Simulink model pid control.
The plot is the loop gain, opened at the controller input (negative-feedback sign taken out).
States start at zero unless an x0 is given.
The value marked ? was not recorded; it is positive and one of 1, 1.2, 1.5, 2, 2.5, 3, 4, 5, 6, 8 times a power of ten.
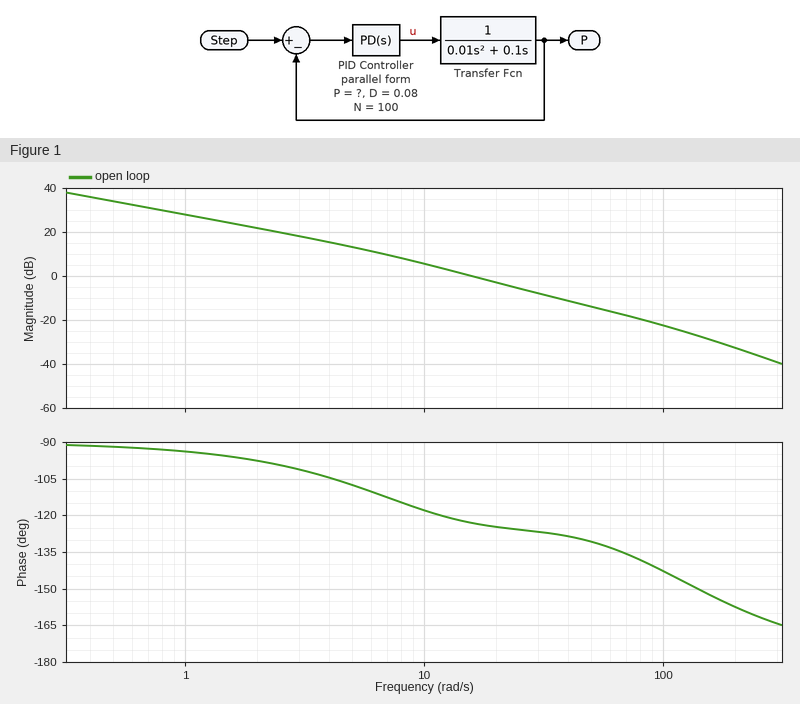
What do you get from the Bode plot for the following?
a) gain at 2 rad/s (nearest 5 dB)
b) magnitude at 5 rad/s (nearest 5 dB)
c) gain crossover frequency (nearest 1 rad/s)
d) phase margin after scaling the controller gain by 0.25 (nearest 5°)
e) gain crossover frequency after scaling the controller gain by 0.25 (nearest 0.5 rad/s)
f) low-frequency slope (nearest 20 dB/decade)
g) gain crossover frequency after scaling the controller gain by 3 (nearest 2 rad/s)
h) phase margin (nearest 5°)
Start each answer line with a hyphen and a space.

- 20 dB
- 15 dB
- 16 rad/s
- 70°
- 5.5 rad/s
- -20 dB/decade
- 34 rad/s
- 55°
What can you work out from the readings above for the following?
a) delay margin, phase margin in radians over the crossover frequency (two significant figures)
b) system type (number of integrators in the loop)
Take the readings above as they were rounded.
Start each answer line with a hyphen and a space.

- 0.060 s
- 1
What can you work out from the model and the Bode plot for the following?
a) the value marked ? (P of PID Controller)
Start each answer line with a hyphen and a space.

- 2.5
